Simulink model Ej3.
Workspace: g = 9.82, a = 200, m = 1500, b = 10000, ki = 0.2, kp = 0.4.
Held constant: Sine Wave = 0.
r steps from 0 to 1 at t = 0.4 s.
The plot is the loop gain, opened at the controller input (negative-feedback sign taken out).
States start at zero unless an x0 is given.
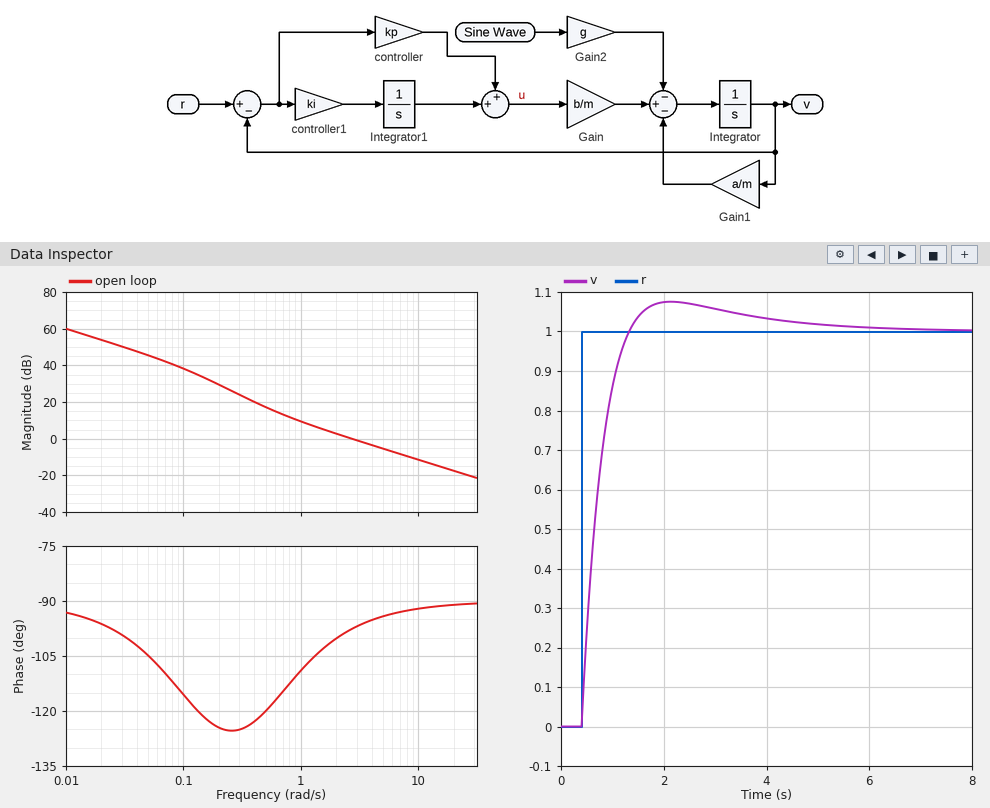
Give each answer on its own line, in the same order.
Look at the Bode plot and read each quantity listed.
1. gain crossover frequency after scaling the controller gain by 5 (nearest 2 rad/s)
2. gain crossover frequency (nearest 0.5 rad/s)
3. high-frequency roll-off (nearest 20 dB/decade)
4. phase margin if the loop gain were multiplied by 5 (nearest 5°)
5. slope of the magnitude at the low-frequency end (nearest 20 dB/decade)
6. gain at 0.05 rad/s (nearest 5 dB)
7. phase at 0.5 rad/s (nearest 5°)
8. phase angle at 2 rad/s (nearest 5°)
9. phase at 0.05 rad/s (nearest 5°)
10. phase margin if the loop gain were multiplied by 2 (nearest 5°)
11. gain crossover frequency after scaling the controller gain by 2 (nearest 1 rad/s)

14 rad/s
2.5 rad/s
-20 dB/decade
90°
-20 dB/decade
45 dB
-120°
-100°
-105°
85°
5 rad/s
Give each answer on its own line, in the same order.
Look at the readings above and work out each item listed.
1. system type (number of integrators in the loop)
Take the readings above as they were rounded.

1
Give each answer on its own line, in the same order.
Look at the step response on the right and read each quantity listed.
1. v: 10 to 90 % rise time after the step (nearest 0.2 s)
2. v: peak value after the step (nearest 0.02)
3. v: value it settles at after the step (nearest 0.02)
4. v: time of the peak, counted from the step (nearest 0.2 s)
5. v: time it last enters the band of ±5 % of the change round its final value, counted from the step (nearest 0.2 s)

0.6 s
1.08
1.00
1.8 s
2.8 s
